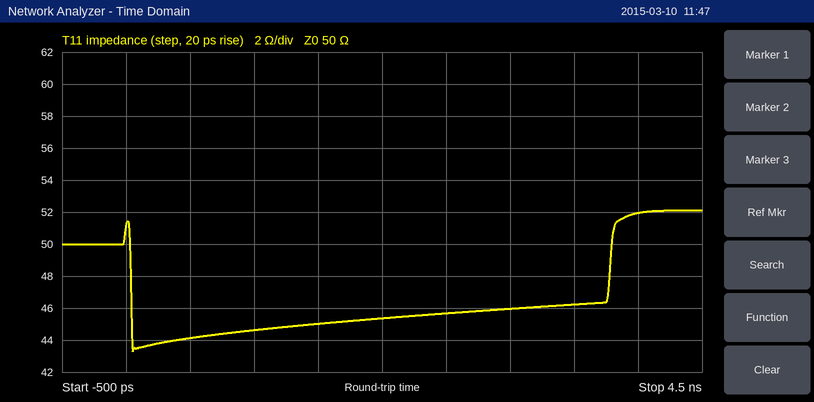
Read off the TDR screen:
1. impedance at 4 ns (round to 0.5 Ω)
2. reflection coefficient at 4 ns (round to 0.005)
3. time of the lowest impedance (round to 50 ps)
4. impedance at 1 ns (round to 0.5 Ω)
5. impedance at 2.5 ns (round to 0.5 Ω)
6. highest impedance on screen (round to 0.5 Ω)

52.0 Ω
+0.020
50 ps
44.5 Ω
45.5 Ω
52.0 Ω
